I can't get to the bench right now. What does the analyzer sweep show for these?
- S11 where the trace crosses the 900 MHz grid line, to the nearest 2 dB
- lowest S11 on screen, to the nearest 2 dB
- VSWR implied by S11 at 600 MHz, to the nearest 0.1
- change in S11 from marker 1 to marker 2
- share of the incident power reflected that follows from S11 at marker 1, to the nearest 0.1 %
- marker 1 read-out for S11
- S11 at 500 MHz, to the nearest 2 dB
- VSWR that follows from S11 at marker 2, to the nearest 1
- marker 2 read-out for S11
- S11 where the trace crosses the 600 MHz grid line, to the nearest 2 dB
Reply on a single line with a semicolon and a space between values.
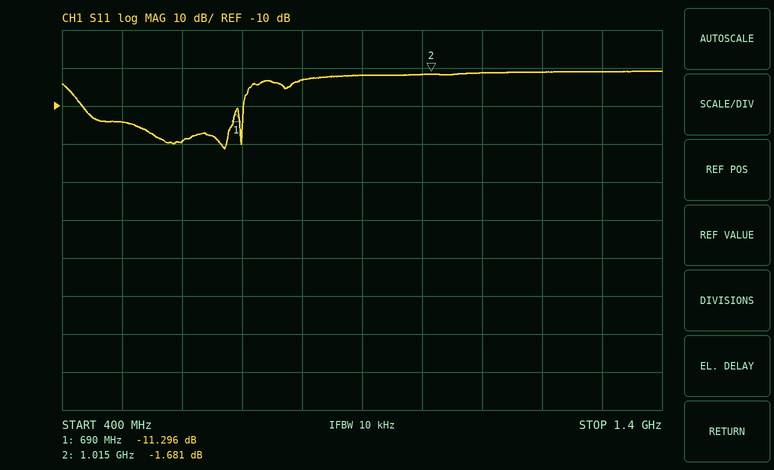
-2 dB; -22 dB; 1.2; 9.615 dB; 7.4 %; -11.296 dB; -14 dB; 10; -1.681 dB; -20 dB
